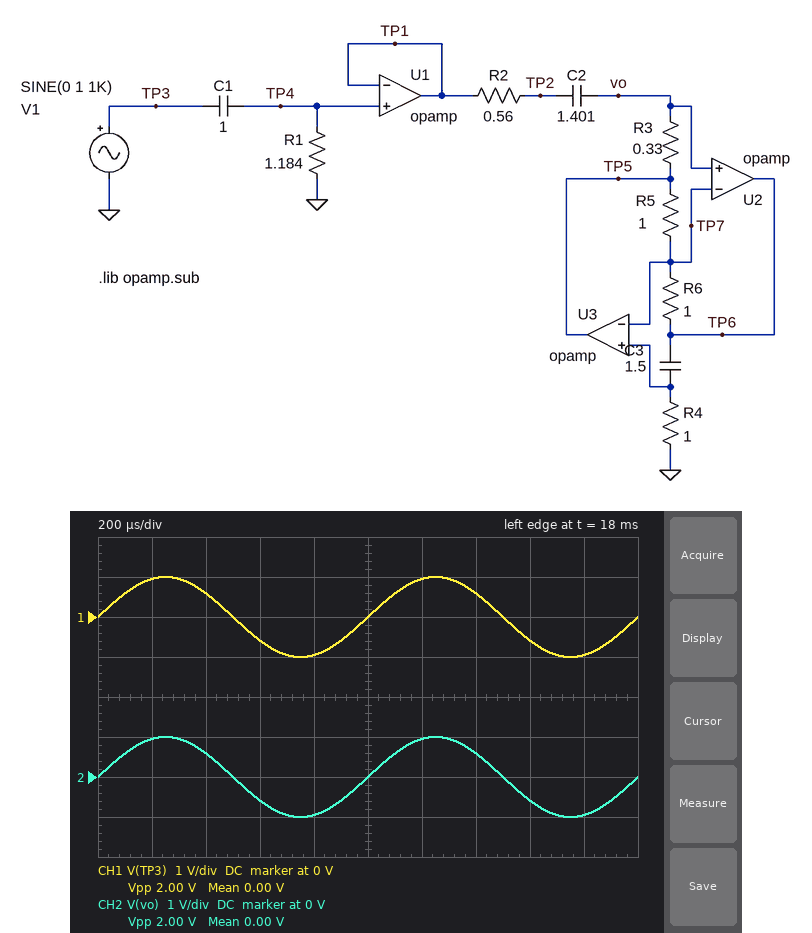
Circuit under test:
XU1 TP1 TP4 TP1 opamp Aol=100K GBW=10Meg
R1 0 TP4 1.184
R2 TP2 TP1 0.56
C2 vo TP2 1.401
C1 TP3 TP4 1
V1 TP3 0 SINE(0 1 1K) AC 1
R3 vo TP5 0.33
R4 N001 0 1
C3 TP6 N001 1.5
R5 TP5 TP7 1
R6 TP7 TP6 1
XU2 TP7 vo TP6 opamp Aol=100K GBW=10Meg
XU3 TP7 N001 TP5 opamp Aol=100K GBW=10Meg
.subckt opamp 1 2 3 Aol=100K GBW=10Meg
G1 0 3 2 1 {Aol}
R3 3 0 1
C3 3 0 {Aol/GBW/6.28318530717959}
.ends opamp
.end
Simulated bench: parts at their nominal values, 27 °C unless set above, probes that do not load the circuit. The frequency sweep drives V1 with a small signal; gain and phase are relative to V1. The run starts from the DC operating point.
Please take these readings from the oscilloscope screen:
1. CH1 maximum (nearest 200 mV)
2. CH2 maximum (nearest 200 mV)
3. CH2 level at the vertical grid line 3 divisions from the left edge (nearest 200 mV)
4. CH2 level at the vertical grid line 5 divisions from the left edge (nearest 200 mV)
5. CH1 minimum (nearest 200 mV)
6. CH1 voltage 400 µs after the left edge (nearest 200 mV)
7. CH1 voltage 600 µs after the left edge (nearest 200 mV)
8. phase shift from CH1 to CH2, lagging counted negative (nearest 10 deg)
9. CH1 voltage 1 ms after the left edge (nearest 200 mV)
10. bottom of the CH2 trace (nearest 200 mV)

1.0 V
1.0 V
-600 mV
0 V
-1.0 V
600 mV
-600 mV
0 deg
0 V
-1.0 V
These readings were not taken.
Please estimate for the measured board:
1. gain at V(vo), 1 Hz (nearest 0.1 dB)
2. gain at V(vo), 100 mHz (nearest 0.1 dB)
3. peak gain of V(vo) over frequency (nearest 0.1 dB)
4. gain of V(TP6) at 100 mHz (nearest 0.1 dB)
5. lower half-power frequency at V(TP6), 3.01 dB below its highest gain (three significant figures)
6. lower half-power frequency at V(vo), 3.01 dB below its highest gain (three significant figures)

0.1 dB
-14.6 dB
0.7 dB
-11.3 dB
166 mHz
176 mHz
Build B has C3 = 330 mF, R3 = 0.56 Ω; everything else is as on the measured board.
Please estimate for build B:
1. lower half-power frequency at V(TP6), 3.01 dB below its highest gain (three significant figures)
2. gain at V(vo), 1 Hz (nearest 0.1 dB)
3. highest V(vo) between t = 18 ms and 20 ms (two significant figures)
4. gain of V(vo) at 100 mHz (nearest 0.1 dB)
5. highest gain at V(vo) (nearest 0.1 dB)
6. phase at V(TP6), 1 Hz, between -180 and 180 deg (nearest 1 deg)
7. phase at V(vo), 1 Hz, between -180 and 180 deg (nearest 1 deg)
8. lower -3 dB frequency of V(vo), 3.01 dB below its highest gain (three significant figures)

216 mHz
-0.3 dB
1.0 V
-24.5 dB
0 dB
10 deg
36 deg
372 mHz
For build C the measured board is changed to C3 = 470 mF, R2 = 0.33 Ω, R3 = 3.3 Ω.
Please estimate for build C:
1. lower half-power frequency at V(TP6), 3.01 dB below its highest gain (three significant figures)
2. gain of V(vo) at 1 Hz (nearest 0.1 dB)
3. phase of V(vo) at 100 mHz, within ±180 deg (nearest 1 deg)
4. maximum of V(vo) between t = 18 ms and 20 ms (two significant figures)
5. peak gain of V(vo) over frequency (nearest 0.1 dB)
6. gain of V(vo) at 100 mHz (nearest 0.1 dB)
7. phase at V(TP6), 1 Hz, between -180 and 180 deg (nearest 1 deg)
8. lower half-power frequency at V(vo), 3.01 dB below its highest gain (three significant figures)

95.2 mHz
0 dB
169 deg
1.0 V
6.3 dB
4.0 dB
-9 deg
98.1 mHz
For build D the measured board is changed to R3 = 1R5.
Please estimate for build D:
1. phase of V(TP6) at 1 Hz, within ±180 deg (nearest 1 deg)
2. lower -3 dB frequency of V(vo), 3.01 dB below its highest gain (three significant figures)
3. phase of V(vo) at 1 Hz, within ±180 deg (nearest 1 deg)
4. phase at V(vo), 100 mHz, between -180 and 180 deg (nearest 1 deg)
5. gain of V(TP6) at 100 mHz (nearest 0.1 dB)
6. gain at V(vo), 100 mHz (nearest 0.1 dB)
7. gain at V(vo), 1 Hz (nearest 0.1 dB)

4 deg
80.9 mHz
10 deg
117 deg
5.9 dB
2.6 dB
0 dB
